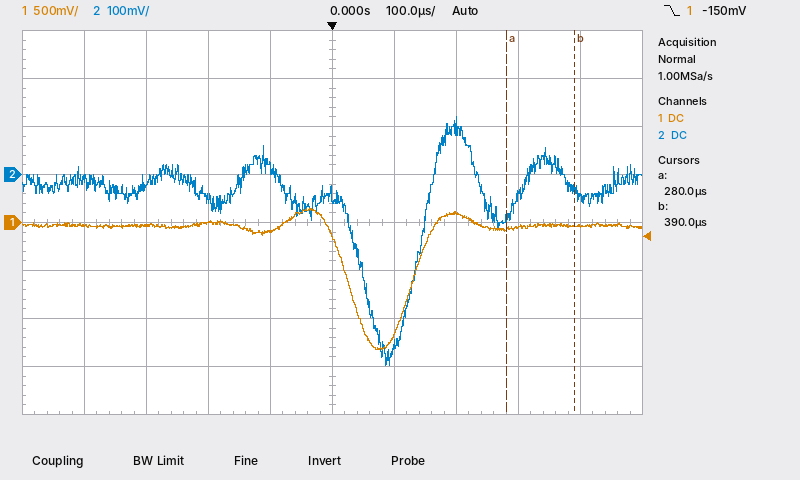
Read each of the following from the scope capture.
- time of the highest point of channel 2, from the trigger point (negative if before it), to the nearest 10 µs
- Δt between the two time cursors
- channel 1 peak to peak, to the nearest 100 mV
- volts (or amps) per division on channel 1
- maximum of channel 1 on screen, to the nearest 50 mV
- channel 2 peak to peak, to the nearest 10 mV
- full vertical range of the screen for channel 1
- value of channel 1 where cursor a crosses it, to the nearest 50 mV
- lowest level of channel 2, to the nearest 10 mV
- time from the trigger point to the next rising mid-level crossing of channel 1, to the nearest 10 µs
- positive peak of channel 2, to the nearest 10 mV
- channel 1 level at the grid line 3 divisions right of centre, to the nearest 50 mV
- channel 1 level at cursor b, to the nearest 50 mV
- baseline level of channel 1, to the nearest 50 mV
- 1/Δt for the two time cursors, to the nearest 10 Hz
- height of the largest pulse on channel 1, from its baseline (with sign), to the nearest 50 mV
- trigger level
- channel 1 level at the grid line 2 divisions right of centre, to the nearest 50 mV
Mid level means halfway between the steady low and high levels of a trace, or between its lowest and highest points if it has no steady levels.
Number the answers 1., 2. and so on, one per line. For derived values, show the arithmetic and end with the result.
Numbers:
1. +200 µs
2. 390 µs − (280 µs) = 110 µs
3. 1.50 V
4. 500 mV
5. 150 mV
6. 120 mV − (-400 mV) = 520 mV
7. 4 V
8. -50 mV
9. -400 mV
10. 130 µs
11. 120 mV
12. -50 mV
13. -50 mV
14. -50 mV
15. 1 / 110 µs ≈ 9.09 kHz
16. -1.30 V
17. -150 mV
18. 100 mV
